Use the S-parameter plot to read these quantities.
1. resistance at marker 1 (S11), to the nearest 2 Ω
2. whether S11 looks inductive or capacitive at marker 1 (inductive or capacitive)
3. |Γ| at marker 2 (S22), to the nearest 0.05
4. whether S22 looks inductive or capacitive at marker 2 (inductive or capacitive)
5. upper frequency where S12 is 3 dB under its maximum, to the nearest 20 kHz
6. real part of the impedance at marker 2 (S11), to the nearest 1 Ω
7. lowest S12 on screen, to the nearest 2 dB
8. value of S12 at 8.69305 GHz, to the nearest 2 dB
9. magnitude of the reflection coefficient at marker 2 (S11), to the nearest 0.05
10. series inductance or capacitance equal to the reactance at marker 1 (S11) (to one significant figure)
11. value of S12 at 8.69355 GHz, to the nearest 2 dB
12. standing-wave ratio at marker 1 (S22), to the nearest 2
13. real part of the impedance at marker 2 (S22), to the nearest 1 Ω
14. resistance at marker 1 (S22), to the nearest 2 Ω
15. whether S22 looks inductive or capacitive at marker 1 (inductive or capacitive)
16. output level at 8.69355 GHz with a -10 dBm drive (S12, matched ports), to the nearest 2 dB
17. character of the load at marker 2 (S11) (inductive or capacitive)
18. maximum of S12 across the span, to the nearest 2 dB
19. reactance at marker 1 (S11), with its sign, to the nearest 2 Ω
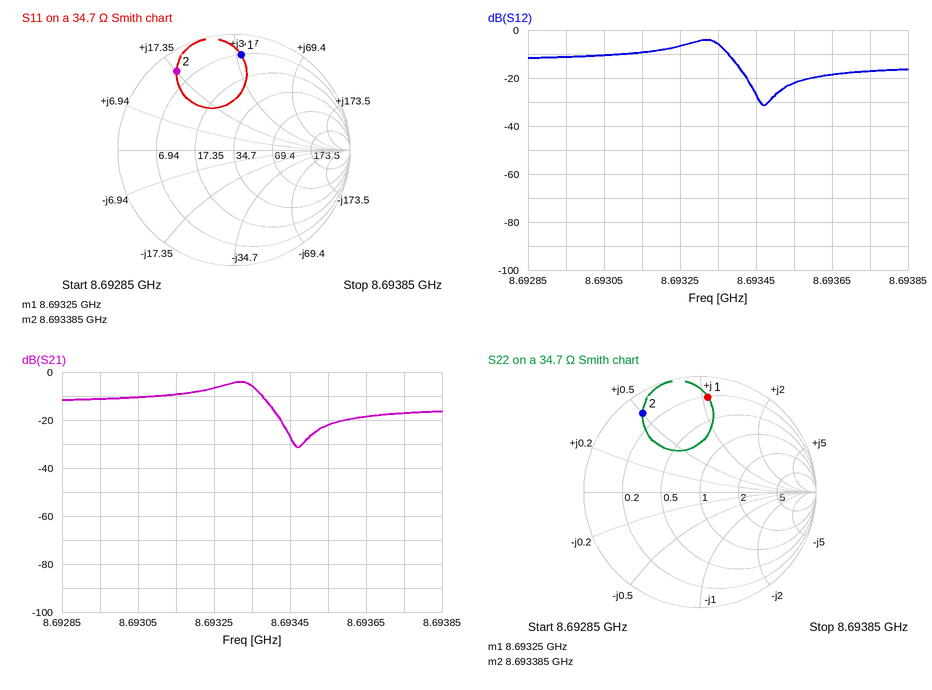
8 Ω
inductive
0.85
inductive
8.69336 GHz
4 Ω
-32 dB
-10 dB
0.85
700 pH
-22 dB
10
4 Ω
8 Ω
inductive
-32 dBm
inductive
-4 dB
+36 Ω
